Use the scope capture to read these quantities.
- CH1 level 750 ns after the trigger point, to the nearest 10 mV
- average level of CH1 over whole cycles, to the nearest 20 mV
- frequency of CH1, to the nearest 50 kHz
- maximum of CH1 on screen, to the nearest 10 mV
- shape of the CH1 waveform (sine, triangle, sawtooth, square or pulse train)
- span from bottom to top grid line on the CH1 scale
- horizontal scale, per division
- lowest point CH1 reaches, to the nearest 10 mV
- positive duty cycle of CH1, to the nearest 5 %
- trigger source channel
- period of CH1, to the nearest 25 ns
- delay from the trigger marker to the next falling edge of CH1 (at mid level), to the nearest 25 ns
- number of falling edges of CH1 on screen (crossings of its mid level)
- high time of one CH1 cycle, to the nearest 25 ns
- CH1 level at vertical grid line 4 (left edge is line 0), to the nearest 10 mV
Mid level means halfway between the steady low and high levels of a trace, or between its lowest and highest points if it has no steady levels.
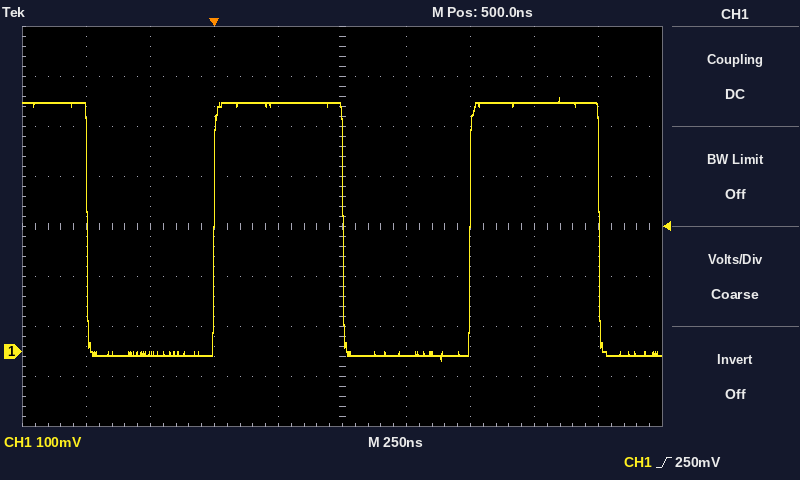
-10 mV
240 mV
1.00 MHz
510 mV
square
800 mV
250 ns
-20 mV
50 %
CH1
1.000 µs
500 ns
3
500 ns
500 mV
